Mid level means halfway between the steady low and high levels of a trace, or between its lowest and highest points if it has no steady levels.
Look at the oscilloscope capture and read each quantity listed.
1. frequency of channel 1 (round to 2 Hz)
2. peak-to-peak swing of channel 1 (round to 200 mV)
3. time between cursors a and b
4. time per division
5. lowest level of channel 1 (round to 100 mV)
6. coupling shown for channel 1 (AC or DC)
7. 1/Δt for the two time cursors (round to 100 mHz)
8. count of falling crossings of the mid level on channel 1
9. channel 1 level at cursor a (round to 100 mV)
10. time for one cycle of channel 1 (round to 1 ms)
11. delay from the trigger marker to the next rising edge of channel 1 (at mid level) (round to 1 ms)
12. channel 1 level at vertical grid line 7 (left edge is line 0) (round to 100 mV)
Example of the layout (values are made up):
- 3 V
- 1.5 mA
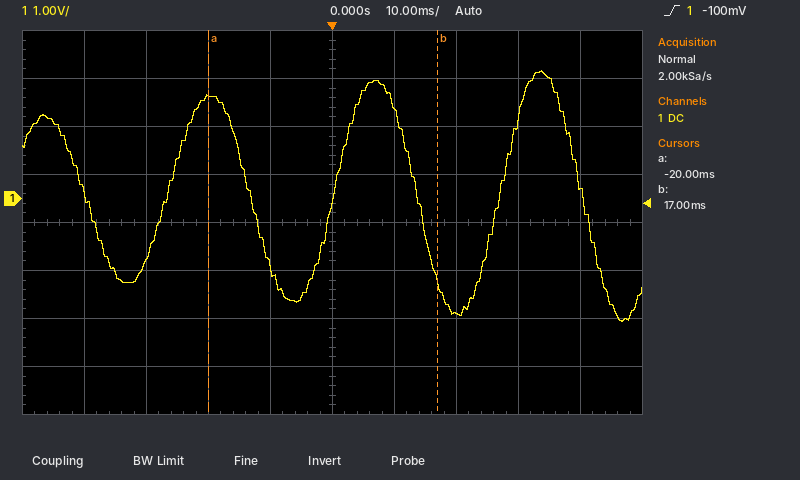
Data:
- 38 Hz
- 5.2 V
- 37 ms
- 10 ms
- -2.6 V
- DC
- 27.0 Hz
- 4
- 2.1 V
- 27 ms
- 27 ms
- -2.4 V
